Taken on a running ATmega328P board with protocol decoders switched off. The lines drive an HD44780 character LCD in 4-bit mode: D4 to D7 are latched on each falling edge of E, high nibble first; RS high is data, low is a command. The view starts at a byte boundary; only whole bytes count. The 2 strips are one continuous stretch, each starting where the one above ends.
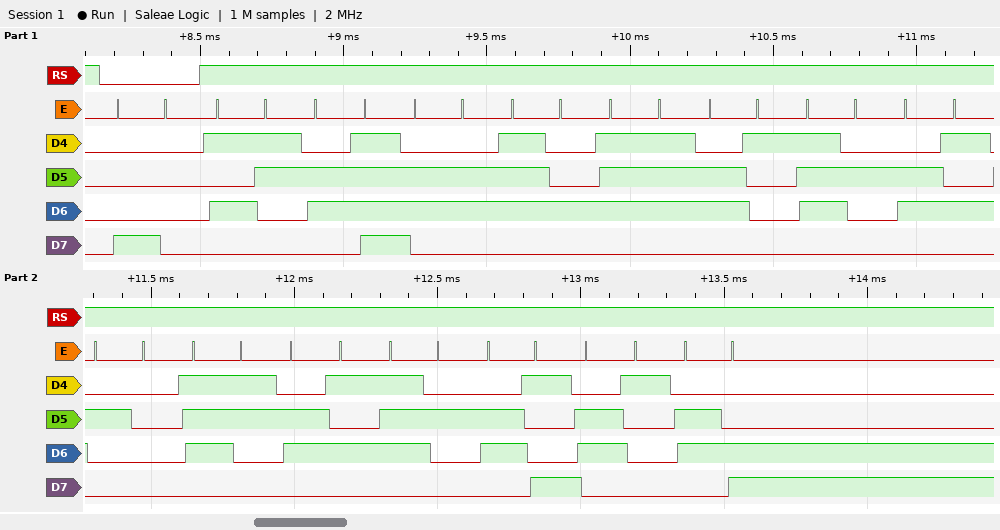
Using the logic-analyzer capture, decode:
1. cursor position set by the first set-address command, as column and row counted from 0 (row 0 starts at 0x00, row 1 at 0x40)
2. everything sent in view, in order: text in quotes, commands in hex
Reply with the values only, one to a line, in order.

column 0, row 0
0x80 "Software serial"
